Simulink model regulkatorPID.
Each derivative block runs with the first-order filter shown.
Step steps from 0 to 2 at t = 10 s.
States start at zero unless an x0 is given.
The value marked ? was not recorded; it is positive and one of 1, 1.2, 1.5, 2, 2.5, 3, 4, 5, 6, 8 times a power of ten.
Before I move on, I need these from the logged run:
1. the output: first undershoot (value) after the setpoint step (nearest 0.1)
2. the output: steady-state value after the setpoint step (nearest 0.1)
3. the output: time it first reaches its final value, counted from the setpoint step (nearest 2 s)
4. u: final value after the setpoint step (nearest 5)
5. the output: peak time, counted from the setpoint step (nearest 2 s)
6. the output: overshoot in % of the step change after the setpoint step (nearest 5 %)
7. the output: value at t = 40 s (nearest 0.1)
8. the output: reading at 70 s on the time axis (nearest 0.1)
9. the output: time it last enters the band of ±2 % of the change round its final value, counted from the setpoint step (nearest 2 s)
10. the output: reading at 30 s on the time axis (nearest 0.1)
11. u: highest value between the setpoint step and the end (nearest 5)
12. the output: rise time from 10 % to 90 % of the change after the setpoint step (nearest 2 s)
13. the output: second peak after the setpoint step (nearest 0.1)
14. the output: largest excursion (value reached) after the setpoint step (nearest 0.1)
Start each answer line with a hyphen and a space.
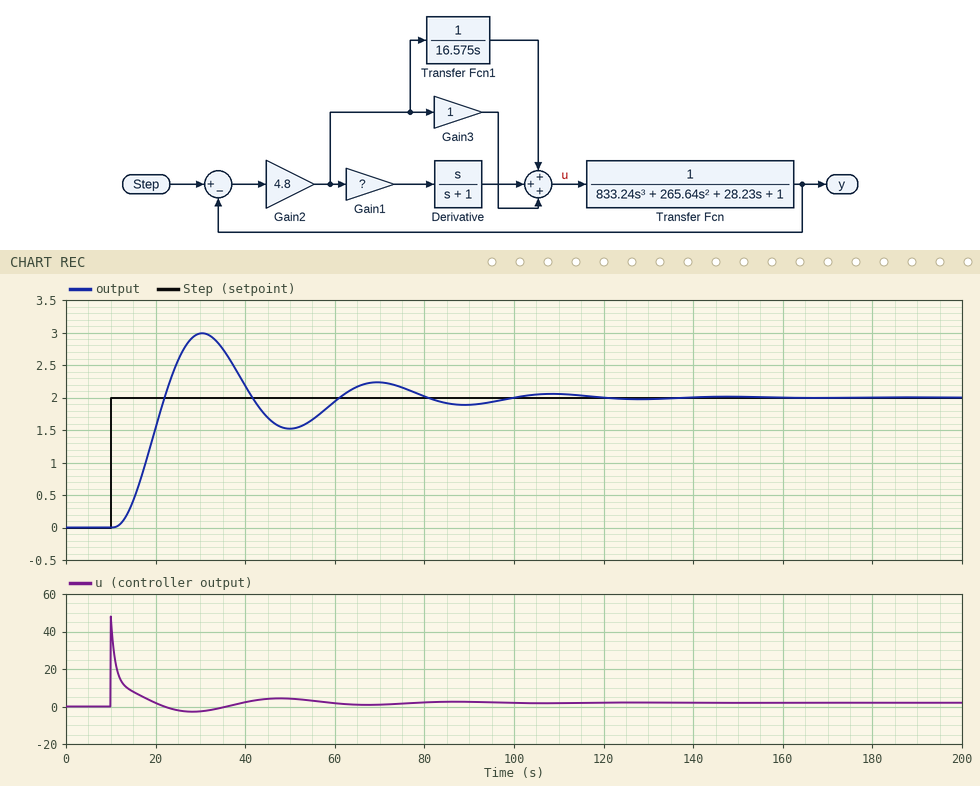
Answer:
- 1.5
- 2.0
- 12 s
- 0
- 20 s
- 50 %
- 2.2
- 2.2
- 104 s
- 3.0
- 50
- 8 s
- 2.2
- 3.0
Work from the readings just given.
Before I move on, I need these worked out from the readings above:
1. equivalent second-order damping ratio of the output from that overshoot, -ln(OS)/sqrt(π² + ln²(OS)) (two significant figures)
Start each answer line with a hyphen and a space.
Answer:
- 0.22
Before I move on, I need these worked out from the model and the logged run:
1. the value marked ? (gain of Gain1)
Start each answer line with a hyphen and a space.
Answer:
- 4
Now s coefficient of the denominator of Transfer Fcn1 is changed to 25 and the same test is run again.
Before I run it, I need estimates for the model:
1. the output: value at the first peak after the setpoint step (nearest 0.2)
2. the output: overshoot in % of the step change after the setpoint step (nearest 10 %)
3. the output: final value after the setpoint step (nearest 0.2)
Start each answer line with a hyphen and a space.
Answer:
- 2.8
- 40 %
- 2.0
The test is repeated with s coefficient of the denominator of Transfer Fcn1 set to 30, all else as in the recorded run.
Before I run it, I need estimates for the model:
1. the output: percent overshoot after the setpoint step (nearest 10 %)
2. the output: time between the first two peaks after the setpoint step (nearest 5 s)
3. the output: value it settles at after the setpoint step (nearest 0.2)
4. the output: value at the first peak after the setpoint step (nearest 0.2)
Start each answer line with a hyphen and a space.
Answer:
- 30 %
- 35 s
- 2.0
- 2.6
